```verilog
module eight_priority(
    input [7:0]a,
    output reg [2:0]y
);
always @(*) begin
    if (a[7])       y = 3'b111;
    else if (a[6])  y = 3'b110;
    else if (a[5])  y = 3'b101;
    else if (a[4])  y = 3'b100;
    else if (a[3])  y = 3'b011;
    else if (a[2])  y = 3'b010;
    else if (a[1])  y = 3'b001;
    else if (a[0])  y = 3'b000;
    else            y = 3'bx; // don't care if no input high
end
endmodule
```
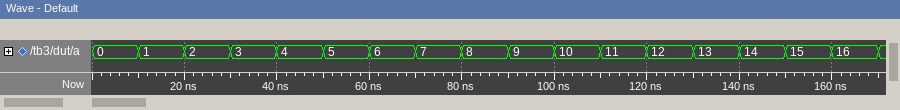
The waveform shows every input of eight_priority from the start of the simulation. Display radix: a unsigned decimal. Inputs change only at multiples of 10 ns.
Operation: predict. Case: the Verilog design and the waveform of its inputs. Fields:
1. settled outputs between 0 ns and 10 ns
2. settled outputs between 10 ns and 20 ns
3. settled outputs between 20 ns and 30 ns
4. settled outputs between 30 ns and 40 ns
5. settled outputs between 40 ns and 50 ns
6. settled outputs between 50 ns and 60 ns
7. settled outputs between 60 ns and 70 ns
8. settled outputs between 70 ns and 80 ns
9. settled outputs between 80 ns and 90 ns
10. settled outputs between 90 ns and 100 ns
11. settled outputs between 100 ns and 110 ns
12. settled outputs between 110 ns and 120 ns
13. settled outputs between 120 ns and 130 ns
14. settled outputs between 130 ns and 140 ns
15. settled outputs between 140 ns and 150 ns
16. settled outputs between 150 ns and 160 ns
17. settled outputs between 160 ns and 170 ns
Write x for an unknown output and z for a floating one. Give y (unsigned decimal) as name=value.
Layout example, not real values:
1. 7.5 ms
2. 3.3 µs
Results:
1. y=x
2. y=0
3. y=1
4. y=1
5. y=2
6. y=2
7. y=2
8. y=2
9. y=3
10. y=3
11. y=3
12. y=3
13. y=3
14. y=3
15. y=3
16. y=3
17. y=4
